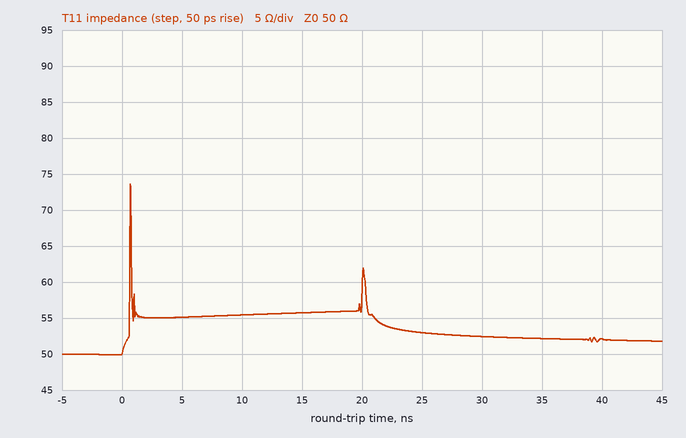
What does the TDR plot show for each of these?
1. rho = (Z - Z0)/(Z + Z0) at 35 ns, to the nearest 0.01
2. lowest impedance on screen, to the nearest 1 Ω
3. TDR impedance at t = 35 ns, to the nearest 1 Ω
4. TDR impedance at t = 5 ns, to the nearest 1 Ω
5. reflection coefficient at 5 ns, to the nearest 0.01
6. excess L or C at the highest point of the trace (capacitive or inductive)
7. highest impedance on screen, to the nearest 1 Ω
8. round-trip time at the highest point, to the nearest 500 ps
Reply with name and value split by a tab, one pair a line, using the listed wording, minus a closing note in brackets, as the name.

rho = (Z - Z0)/(Z + Z0) at 35 ns, to the nearest 0.01	+0.02
lowest impedance on screen, to the nearest 1 Ω	50 Ω
TDR impedance at t = 35 ns, to the nearest 1 Ω	52 Ω
TDR impedance at t = 5 ns, to the nearest 1 Ω	55 Ω
reflection coefficient at 5 ns, to the nearest 0.01	+0.05
excess L or C at the highest point of the trace	inductive
highest impedance on screen, to the nearest 1 Ω	74 Ω
round-trip time at the highest point, to the nearest 500 ps	500 ps
